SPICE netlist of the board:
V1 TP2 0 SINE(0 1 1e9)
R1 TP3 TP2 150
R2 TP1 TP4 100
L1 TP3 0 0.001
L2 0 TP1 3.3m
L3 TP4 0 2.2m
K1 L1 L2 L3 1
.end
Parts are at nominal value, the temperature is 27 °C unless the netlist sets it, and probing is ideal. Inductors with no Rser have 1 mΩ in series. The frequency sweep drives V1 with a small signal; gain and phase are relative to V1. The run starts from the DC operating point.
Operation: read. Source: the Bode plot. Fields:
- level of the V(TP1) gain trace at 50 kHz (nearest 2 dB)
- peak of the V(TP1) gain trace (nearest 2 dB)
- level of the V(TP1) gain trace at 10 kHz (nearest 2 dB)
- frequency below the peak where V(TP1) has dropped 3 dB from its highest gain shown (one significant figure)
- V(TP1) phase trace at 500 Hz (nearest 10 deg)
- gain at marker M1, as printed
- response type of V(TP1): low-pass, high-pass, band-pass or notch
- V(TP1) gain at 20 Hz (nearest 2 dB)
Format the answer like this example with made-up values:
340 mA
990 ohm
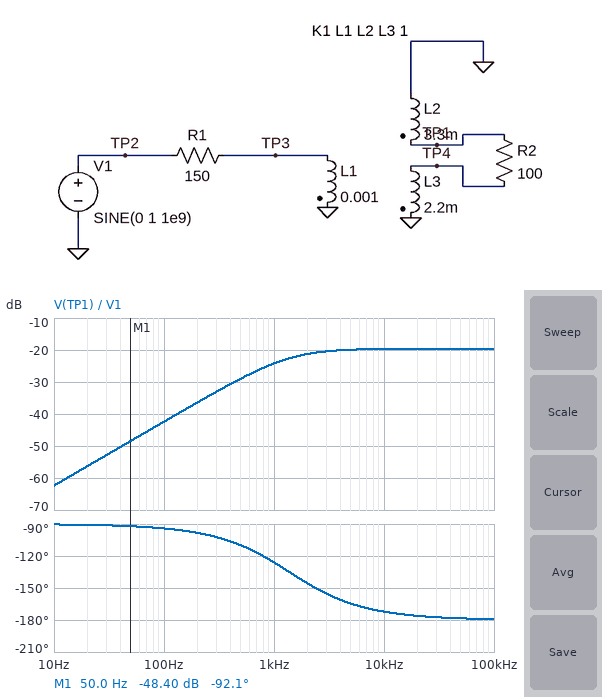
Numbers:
-20 dB
-20 dB
-20 dB
1 kHz
-110 deg
-48.40 dB
high-pass
-56 dB
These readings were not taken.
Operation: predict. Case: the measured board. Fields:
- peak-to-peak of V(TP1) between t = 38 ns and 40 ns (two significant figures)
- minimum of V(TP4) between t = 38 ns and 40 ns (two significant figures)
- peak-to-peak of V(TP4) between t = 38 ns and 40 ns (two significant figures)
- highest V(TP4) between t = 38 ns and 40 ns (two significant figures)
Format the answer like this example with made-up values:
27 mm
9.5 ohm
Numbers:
210 mV
-86 mV
170 mV
86 mV
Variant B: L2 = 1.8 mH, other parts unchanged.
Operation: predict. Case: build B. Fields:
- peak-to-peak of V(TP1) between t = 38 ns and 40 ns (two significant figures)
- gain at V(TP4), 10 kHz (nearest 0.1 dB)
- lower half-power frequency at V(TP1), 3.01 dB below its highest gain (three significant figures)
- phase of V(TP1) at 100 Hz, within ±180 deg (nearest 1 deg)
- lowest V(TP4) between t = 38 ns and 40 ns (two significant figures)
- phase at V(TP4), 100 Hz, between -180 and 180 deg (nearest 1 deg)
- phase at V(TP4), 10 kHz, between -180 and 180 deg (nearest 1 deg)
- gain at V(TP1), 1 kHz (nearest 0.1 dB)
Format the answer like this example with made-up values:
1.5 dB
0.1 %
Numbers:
210 mV
-19.0 dB
1.84 kHz
-93 deg
-110 mV
87 deg
10 deg
-26.1 dB
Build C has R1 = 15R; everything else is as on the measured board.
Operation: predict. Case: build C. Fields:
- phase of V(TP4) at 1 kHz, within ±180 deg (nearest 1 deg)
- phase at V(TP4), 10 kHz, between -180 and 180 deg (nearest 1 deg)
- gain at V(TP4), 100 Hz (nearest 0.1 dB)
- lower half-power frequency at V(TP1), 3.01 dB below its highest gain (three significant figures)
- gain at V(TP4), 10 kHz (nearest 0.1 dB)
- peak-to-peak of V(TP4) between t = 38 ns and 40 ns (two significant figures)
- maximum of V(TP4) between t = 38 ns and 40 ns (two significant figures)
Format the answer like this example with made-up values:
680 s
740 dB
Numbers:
42 deg
5 deg
-24.2 dB
907 Hz
-5.0 dB
1.1 V
560 mV
